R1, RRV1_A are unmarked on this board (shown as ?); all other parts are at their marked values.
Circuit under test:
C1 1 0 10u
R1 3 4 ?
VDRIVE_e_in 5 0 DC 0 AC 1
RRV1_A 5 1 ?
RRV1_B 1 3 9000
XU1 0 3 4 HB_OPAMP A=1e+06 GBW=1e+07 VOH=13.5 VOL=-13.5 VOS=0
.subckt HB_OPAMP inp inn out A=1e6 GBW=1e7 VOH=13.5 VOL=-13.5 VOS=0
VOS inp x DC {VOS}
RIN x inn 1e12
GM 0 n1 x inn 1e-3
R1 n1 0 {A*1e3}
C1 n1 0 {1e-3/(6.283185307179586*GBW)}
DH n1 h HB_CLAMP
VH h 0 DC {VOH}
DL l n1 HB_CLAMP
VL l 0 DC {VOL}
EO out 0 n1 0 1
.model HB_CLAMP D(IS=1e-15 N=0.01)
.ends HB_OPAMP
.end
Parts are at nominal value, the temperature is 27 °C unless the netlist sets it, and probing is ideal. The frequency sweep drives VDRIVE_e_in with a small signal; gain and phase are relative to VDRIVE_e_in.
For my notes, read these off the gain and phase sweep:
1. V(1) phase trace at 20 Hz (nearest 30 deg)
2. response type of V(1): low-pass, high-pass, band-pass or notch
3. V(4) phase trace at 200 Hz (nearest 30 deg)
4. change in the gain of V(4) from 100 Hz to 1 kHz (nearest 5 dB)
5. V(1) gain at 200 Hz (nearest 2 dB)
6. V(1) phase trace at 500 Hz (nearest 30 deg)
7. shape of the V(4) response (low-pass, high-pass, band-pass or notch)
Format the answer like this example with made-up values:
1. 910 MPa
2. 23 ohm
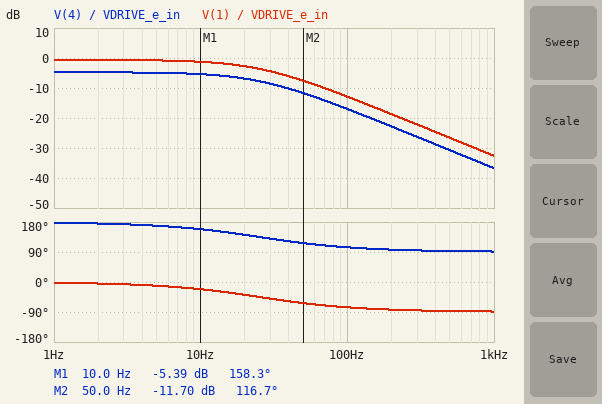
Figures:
1. -30 deg
2. low-pass
3. 90 deg
4. -20 dB
5. -18 dB
6. -90 deg
7. low-pass
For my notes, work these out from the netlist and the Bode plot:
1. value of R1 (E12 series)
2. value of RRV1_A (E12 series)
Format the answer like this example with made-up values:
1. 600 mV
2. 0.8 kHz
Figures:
1. 5.6 kΩ
2. 680 Ω
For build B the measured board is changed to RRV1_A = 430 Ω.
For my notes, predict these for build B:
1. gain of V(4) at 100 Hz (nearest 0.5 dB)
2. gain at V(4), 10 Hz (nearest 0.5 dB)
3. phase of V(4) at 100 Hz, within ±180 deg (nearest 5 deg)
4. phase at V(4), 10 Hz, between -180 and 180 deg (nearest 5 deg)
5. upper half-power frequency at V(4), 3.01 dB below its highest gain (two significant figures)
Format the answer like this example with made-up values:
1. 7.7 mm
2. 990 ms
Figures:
1. -13.5 dB
2. -5.0 dB
3. 110 deg
4. 165 deg
5. 39 Hz
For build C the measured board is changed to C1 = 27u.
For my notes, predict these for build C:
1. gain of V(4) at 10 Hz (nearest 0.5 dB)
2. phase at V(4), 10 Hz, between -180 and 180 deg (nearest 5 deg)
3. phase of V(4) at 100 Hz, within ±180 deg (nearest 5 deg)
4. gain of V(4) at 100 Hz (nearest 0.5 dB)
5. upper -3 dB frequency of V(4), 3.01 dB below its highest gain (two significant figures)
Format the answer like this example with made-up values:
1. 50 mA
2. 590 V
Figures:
1. -8.0 dB
2. 135 deg
3. 95 deg
4. -25.5 dB
5. 9.3 Hz
